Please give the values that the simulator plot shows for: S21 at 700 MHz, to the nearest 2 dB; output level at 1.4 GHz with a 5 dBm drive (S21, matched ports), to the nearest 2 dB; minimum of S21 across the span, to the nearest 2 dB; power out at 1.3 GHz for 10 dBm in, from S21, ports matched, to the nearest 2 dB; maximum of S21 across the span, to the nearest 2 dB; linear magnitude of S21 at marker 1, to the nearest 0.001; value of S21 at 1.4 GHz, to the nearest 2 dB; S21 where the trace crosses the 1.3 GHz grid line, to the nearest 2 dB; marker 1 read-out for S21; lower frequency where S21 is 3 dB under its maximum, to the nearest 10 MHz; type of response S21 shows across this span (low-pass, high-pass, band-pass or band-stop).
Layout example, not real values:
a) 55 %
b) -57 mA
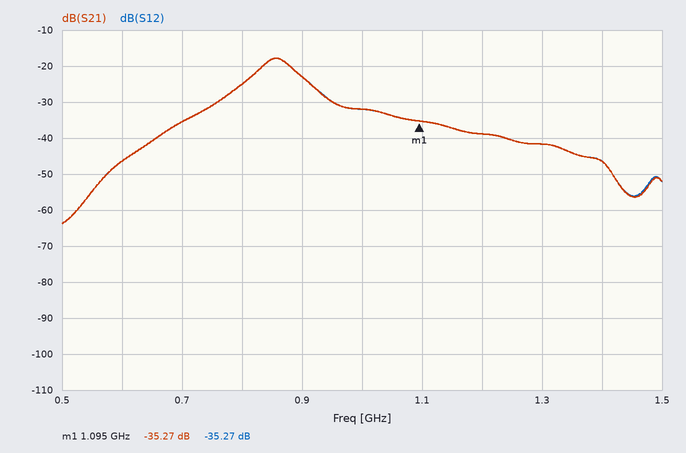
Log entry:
a) -36 dB
b) -42 dBm
c) -64 dB
d) -32 dBm
e) -18 dB
f) 0.017
g) -46 dB
h) -42 dB
i) -35.27 dB
j) 830 MHz
k) band-pass
